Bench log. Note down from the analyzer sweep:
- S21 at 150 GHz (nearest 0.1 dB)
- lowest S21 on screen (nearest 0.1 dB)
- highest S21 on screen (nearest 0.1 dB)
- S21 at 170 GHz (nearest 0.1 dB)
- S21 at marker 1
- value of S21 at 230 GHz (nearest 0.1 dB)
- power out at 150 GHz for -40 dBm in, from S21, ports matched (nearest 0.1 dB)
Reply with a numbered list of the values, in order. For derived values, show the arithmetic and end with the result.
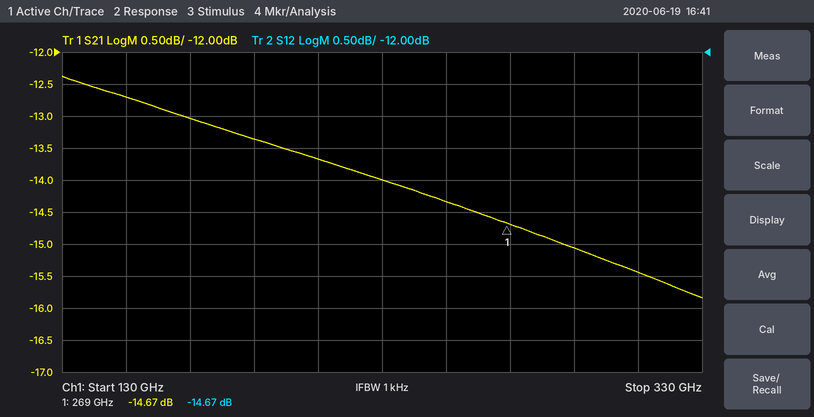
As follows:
1. -12.7 dB
2. -15.8 dB
3. -12.4 dB
4. -13.0 dB
5. -14.67 dB
6. -14.0 dB
7. -40 dBm + (-12.7 dB) = -52.7 dBm
